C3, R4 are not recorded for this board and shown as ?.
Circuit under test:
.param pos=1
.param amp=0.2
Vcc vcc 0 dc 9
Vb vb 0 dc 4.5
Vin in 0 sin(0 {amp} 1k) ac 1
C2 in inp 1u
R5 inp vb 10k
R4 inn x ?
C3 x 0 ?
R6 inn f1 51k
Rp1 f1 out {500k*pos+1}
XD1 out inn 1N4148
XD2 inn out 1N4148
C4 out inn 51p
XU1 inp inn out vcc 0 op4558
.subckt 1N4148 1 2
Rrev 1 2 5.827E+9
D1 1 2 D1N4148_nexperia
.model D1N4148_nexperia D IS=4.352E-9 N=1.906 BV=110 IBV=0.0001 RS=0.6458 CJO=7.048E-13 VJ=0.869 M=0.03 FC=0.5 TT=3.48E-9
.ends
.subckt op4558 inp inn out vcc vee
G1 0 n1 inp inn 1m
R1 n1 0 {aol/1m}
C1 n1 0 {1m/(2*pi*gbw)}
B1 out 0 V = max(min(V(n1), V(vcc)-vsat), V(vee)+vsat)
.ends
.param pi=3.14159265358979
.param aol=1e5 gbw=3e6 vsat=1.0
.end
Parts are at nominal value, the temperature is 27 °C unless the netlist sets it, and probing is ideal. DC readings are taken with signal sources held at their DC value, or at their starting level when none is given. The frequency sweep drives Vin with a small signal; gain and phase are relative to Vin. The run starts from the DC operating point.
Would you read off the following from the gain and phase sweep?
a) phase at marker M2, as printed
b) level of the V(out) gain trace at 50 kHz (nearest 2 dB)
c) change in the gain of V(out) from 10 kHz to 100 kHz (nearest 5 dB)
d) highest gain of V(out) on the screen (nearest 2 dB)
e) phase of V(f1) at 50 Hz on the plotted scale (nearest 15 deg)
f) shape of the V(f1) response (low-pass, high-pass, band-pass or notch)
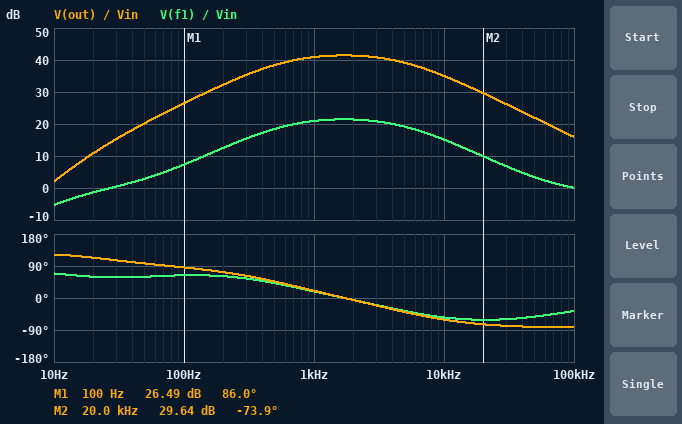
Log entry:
-73.9 deg
22 dB
-20 dB
42 dB
60 deg
band-pass
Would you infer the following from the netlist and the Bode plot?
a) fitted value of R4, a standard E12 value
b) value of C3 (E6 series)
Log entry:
3.9 kΩ
68 nF
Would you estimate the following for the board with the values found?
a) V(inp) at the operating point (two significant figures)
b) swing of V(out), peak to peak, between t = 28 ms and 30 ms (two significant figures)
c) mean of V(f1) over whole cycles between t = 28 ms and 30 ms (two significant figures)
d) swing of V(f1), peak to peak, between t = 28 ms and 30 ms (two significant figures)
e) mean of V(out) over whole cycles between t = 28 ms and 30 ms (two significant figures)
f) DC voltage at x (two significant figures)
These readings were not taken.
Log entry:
4.5 V
1.3 V
4.5 V
480 mV
4.5 V
4.5 V
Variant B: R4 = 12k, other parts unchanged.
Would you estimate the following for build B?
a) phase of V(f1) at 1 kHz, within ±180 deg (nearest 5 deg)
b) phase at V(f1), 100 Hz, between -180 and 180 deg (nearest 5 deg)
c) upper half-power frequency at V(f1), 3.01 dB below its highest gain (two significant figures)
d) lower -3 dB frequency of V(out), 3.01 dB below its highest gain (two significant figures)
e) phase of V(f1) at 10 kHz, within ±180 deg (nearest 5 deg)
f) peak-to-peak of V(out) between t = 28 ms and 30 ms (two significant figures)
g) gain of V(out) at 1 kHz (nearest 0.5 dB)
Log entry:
0 deg
50 deg
6.2 kHz
180 Hz
-40 deg
1.2 V
32.5 dB
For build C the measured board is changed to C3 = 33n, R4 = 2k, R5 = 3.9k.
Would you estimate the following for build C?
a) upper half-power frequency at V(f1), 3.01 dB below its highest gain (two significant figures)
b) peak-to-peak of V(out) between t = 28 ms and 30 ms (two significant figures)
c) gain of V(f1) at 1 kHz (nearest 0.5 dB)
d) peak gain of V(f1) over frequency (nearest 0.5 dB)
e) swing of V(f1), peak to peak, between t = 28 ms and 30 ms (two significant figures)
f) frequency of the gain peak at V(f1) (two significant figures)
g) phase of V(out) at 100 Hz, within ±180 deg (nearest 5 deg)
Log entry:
7.0 kHz
1.2 V
19.5 dB
25.0 dB
470 mV
3.1 kHz
105 deg
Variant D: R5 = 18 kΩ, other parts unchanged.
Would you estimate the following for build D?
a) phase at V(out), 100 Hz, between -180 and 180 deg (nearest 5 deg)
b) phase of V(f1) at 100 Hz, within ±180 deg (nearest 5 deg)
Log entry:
80 deg
60 deg
